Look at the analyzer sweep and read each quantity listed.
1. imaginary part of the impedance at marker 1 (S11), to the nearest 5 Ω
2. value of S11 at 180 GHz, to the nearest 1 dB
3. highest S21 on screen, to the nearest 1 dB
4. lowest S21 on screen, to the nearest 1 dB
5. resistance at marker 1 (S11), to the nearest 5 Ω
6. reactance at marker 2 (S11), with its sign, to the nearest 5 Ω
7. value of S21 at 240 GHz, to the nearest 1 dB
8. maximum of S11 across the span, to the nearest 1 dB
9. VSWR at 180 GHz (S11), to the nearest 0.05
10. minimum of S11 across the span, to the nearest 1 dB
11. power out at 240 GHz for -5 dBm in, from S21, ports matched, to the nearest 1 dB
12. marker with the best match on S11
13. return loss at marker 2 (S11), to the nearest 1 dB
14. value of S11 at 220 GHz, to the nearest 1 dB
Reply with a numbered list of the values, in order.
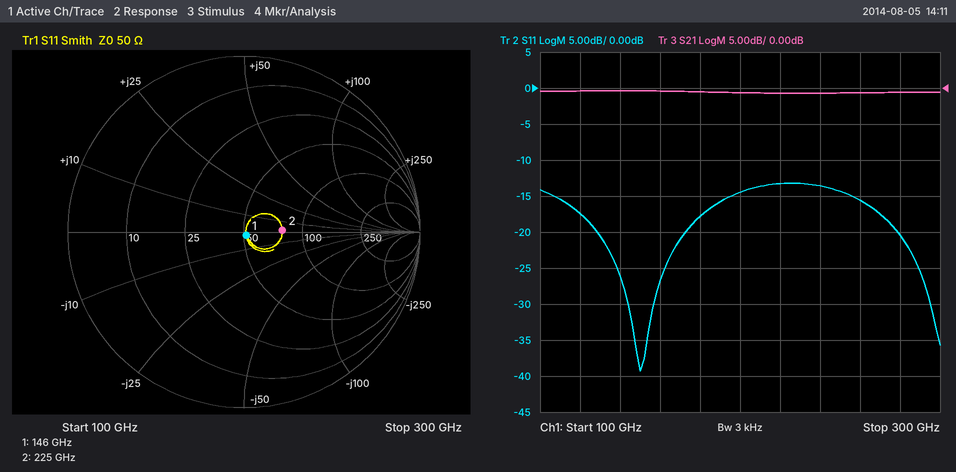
1. 0 Ω
2. -18 dB
3. 0 dB
4. -1 dB
5. 50 Ω
6. 0 Ω
7. -1 dB
8. -13 dB
9. 1.30
10. -39 dB
11. -6 dBm
12. marker 1
13. 13 dB
14. -13 dB
